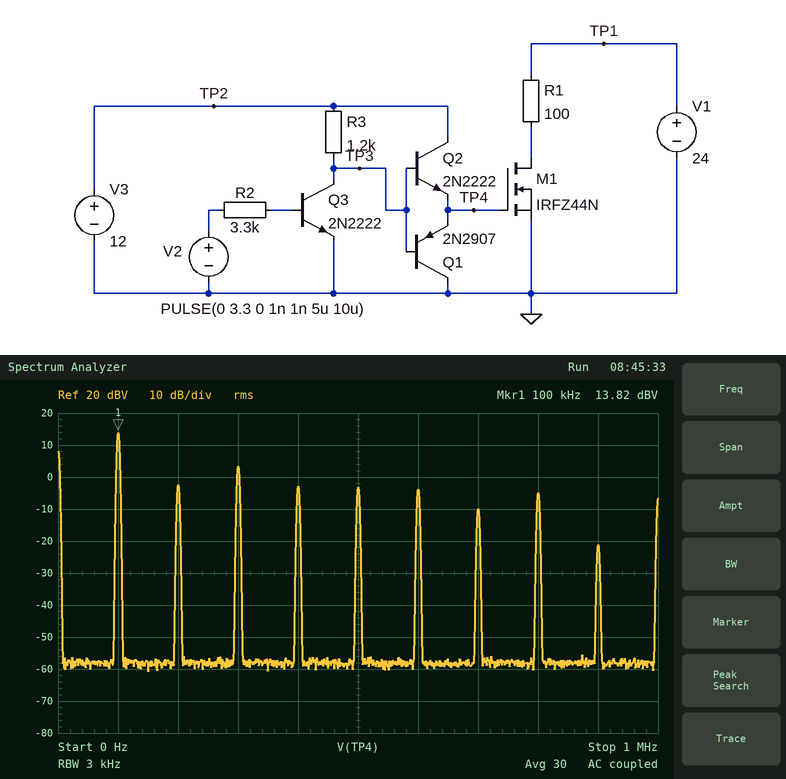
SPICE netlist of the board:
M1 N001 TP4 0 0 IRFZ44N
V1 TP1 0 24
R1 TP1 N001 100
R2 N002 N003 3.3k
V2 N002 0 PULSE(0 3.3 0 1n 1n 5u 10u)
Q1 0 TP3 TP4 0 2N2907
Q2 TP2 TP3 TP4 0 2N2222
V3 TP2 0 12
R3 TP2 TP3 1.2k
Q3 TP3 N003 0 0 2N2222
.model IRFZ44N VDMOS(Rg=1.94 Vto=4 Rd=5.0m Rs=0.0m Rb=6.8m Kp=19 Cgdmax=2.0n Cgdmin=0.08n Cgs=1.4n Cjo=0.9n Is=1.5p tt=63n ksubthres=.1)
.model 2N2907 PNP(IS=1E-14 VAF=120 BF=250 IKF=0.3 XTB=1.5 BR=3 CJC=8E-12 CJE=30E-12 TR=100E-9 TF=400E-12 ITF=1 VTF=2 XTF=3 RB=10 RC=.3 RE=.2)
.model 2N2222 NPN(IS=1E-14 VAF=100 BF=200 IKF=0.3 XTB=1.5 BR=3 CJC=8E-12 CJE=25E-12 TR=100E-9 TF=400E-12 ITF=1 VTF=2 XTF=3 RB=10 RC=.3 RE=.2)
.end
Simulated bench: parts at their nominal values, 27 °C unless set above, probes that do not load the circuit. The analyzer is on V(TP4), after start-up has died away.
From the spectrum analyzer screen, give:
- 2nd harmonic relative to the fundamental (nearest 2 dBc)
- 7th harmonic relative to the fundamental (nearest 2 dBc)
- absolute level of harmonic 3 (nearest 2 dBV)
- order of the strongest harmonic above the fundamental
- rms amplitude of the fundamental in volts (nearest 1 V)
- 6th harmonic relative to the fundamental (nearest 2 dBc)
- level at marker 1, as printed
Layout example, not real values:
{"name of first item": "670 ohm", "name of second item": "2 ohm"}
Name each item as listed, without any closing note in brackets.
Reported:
{"2nd harmonic relative to the fundamental": "-16 dBc", "7th harmonic relative to the fundamental": "-24 dBc", "absolute level of harmonic 3": "4 dBV", "order of the strongest harmonic above the fundamental": "3", "rms amplitude of the fundamental in volts": "5 V", "6th harmonic relative to the fundamental": "-18 dBc", "level at marker 1, as printed": "13.82 dBV"}
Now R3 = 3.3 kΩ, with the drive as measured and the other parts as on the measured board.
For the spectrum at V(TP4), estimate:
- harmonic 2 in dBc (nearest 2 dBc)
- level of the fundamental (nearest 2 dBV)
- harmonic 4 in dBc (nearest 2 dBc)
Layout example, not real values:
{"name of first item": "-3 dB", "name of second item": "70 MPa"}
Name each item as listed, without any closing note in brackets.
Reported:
{"harmonic 2 in dBc": "-14 dBc", "level of the fundamental": "14 dBV", "harmonic 4 in dBc": "-16 dBc"}
